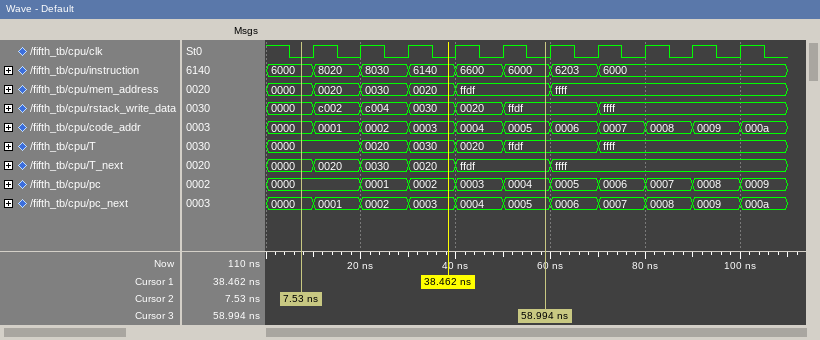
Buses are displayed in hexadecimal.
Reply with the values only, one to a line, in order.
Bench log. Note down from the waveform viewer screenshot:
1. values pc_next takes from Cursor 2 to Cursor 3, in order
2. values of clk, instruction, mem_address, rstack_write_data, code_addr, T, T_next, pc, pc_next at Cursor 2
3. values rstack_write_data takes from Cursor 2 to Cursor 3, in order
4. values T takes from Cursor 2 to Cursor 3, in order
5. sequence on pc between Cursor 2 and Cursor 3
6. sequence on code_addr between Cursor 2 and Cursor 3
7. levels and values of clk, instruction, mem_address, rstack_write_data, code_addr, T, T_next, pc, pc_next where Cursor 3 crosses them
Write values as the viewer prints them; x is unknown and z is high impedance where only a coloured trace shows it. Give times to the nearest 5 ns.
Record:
0000, 0001, 0002, 0003, 0004, 0005
clk=0, instruction=6000, mem_address=0000, rstack_write_data=0000, code_addr=0000, T=0000, T_next=0000, pc=0000, pc_next=0000
0000, c002, c004, 0030, 0020, ffdf
0000, 0020, 0030, 0020, ffdf
0000, 0001, 0002, 0003, 0004
0000, 0001, 0002, 0003, 0004, 0005
clk=0, instruction=6000, mem_address=ffdf, rstack_write_data=ffdf, code_addr=0005, T=ffdf, T_next=ffdf, pc=0004, pc_next=0005
